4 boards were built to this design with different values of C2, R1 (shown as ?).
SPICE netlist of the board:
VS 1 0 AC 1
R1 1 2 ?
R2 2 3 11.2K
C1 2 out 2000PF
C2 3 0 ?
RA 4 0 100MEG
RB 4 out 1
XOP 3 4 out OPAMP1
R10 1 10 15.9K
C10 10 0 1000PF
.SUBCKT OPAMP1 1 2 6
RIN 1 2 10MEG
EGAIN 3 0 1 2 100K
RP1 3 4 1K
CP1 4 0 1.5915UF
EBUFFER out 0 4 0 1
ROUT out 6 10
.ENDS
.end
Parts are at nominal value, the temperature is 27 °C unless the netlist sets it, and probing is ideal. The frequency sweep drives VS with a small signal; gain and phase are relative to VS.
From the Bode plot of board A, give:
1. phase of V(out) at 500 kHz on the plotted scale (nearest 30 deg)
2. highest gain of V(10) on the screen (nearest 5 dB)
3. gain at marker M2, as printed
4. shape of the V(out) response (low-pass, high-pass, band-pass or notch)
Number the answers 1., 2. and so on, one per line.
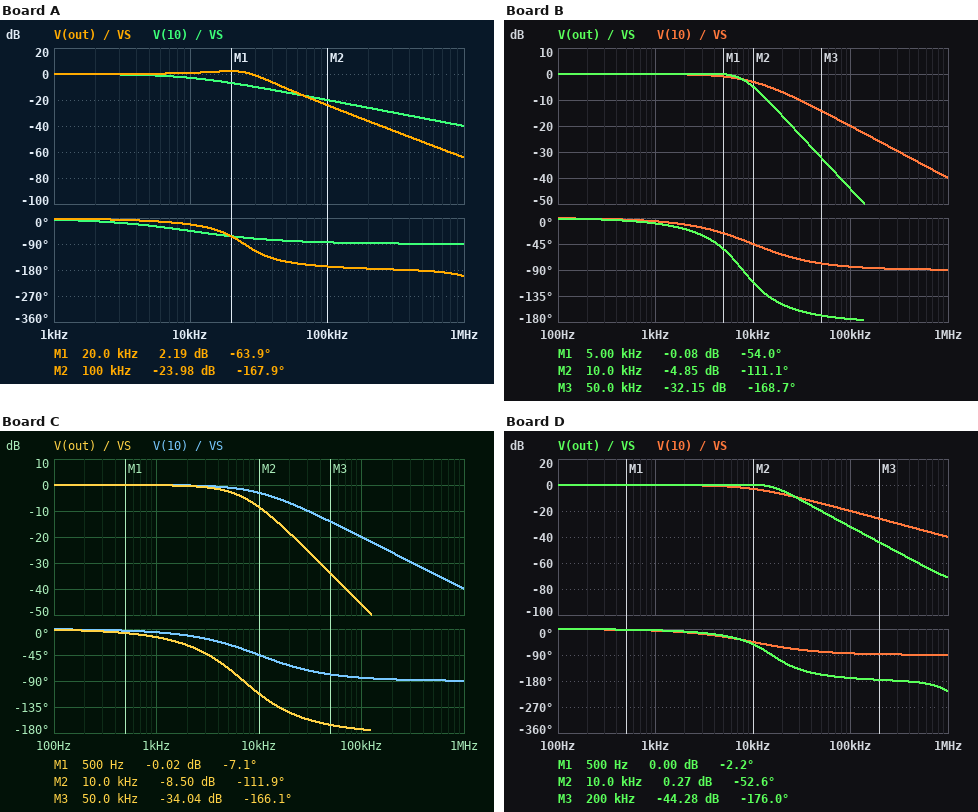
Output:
1. -180 deg
2. 0 dB
3. -23.98 dB
4. low-pass
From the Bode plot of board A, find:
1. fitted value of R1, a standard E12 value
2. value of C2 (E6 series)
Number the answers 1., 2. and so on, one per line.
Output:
1. 5.6 kΩ
2. 330 pF
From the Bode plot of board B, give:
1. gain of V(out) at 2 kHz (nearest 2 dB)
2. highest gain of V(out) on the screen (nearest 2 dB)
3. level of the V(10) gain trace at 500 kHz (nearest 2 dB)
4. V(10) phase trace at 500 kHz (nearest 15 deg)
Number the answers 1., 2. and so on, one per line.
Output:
1. 0 dB
2. 0 dB
3. -34 dB
4. -90 deg
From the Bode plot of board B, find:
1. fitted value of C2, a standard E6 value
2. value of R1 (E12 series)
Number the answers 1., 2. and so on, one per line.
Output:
1. 680 pF
2. 27 kΩ
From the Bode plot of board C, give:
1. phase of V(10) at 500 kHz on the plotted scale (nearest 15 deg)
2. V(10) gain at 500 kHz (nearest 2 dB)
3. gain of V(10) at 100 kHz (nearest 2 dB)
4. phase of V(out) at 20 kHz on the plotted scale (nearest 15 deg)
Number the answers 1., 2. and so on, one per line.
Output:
1. -90 deg
2. -34 dB
3. -20 dB
4. -150 deg
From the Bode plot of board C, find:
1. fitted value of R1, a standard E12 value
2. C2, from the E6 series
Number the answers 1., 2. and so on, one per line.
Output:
1. 15 kΩ
2. 1.5 nF
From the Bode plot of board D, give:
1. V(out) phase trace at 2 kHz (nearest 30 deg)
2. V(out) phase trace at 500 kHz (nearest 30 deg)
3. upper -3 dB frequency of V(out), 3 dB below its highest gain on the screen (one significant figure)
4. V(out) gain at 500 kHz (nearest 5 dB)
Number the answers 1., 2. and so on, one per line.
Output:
1. 0 deg
2. -180 deg
3. 20 kHz
4. -60 dB
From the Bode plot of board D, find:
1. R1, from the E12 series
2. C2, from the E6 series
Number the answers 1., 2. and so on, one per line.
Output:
1. 6.8 kΩ
2. 680 pF
